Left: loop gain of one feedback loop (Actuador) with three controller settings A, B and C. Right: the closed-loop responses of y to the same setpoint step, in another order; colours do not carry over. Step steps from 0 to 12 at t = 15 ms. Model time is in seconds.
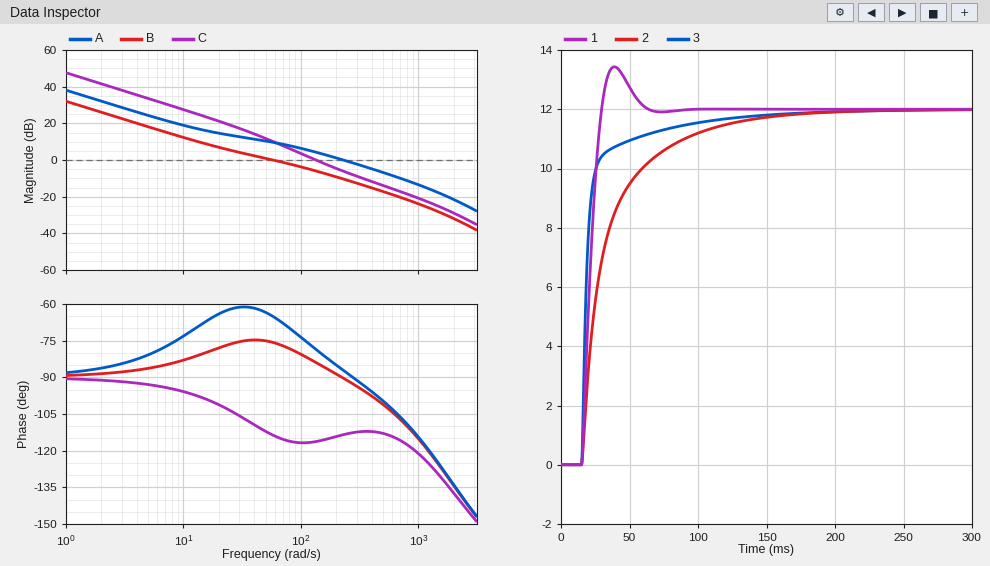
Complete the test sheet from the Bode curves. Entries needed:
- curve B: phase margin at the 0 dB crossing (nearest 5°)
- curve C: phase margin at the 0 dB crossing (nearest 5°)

105°
65°
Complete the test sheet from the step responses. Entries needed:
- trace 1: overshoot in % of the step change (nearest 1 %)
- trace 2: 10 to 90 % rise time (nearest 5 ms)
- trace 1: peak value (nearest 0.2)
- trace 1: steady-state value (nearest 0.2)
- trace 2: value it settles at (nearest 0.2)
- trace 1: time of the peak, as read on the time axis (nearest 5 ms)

12 %
65 ms
13.4
12.0
12.0
40 ms
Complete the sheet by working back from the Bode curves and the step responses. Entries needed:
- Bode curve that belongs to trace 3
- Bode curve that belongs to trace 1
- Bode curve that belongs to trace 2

A
C
B
